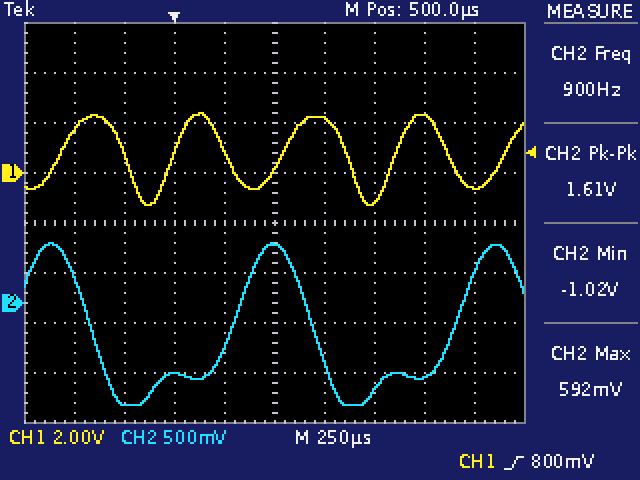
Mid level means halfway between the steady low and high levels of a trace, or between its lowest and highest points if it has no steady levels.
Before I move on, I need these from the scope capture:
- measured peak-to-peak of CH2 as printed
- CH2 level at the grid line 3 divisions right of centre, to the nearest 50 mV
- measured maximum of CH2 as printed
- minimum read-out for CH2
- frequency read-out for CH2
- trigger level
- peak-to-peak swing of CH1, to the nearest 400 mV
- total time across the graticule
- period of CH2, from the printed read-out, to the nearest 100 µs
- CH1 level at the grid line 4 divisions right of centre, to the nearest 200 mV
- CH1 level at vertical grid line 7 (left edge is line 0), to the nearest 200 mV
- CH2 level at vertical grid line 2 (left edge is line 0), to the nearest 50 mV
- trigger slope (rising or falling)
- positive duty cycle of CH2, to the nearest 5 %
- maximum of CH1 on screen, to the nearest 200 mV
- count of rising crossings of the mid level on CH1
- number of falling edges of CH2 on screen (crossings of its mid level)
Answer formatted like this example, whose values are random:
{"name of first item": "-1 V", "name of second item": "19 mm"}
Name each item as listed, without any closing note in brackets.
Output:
{"measured peak-to-peak of CH2 as printed": "1.61 V", "CH2 level at the grid line 3 divisions right of centre, to the nearest 50 mV": "-750 mV", "measured maximum of CH2 as printed": "592 mV", "minimum read-out for CH2": "-1.02 V", "frequency read-out for CH2": "900 Hz", "trigger level": "800 mV", "peak-to-peak swing of CH1, to the nearest 400 mV": "3.6 V", "total time across the graticule": "2.5 ms", "period of CH2, from the printed read-out, to the nearest 100 µs": "1.1 ms", "CH1 level at the grid line 4 divisions right of centre, to the nearest 200 mV": "-600 mV", "CH1 level at vertical grid line 7 (left edge is line 0), to the nearest 200 mV": "-1.2 V", "CH2 level at vertical grid line 2 (left edge is line 0), to the nearest 50 mV": "-1.00 V", "trigger slope": "rising", "positive duty cycle of CH2, to the nearest 5 %": "35 %", "maximum of CH1 on screen, to the nearest 200 mV": "2.4 V", "count of rising crossings of the mid level on CH1": "5", "number of falling edges of CH2 on screen": "2"}
